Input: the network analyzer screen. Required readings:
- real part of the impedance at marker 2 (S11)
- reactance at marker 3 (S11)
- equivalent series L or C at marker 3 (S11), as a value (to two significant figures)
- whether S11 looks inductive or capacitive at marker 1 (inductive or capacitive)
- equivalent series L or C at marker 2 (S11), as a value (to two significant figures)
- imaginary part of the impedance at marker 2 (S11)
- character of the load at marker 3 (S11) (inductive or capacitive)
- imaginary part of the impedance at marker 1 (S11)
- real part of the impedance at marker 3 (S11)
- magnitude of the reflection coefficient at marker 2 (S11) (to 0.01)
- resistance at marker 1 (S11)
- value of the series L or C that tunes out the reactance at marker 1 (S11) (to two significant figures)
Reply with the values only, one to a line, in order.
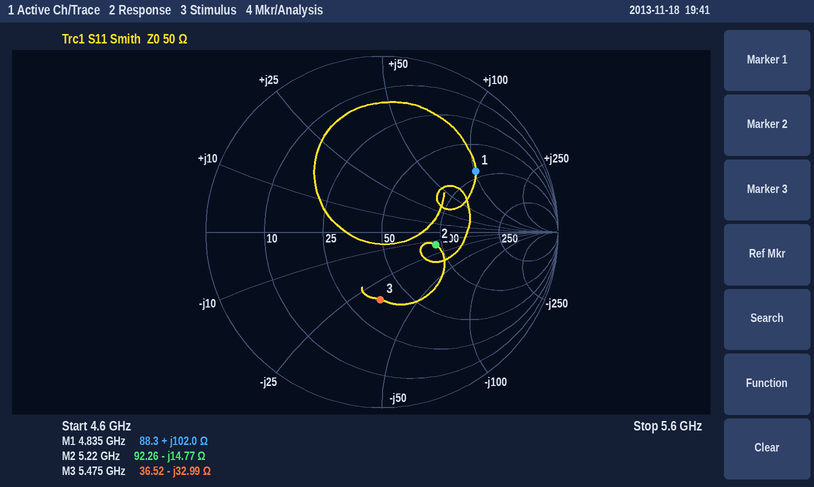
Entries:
92.26 Ω
-32.99 Ω
880 fF
inductive
2.1 pF
-14.77 Ω
capacitive
+102.0 Ω
36.52 Ω
0.31
88.3 Ω
320 fF
